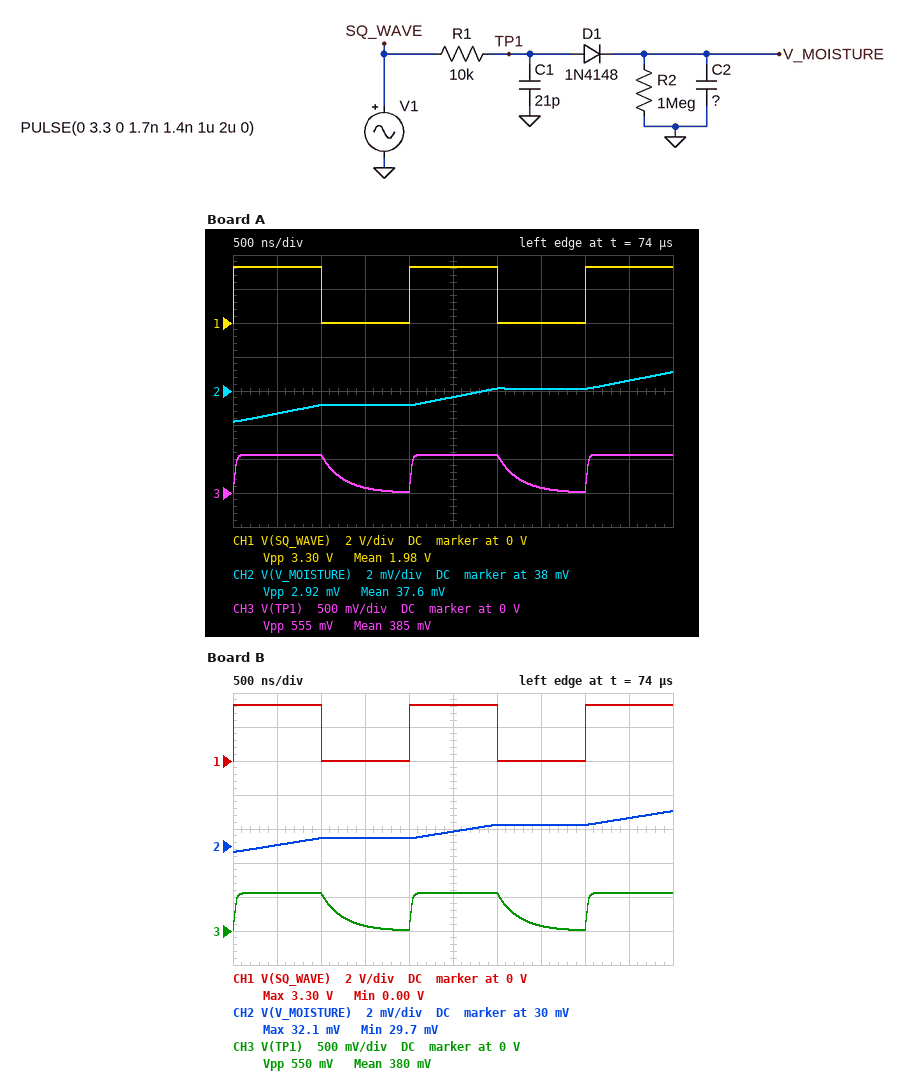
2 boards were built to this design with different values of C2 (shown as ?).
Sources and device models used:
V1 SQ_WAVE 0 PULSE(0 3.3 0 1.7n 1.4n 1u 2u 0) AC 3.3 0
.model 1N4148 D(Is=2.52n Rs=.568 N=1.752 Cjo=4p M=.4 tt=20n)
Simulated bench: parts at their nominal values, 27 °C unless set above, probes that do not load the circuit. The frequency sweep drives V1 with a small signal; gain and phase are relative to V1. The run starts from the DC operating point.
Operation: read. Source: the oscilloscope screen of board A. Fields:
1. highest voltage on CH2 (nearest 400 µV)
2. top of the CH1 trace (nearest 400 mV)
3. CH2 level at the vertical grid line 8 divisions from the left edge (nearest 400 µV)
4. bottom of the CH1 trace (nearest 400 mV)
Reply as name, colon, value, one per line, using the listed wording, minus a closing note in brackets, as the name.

highest voltage on CH2: 39.2 mV
top of the CH1 trace: 3.2 V
CH2 level at the vertical grid line 8 divisions from the left edge: 38.0 mV
bottom of the CH1 trace: 0 V
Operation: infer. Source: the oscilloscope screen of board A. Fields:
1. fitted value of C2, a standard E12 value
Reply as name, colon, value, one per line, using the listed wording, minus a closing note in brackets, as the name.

fitted value of C2, a standard E12 value: 270 nF
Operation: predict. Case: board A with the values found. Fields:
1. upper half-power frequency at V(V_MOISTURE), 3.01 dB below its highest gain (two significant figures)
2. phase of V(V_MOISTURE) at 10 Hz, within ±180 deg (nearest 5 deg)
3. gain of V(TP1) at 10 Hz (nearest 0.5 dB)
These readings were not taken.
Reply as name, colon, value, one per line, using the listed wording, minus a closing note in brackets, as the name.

upper half-power frequency at V(V_MOISTURE), 3.01 dB below its highest gain: 620 mHz
phase of V(V_MOISTURE) at 10 Hz, within ±180 deg: -85 deg
gain of V(TP1) at 10 Hz: 0 dB
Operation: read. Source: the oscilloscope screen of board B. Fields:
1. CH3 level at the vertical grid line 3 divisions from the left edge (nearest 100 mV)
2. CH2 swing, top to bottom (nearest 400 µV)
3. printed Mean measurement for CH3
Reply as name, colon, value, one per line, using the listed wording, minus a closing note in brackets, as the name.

CH3 level at the vertical grid line 3 divisions from the left edge: 100 mV
CH2 swing, top to bottom: 2.4 mV
printed Mean measurement for CH3: 380 mV
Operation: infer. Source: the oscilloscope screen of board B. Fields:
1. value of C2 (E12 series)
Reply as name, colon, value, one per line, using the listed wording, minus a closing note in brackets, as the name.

value of C2: 330 nF
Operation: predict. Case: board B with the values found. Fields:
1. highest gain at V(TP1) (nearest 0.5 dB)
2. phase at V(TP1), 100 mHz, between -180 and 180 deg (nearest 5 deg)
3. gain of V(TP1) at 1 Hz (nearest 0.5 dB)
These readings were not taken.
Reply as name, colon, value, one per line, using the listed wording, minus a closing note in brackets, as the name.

highest gain at V(TP1): 0 dB
phase at V(TP1), 100 mHz, between -180 and 180 deg: 0 deg
gain of V(TP1) at 1 Hz: 0 dB
